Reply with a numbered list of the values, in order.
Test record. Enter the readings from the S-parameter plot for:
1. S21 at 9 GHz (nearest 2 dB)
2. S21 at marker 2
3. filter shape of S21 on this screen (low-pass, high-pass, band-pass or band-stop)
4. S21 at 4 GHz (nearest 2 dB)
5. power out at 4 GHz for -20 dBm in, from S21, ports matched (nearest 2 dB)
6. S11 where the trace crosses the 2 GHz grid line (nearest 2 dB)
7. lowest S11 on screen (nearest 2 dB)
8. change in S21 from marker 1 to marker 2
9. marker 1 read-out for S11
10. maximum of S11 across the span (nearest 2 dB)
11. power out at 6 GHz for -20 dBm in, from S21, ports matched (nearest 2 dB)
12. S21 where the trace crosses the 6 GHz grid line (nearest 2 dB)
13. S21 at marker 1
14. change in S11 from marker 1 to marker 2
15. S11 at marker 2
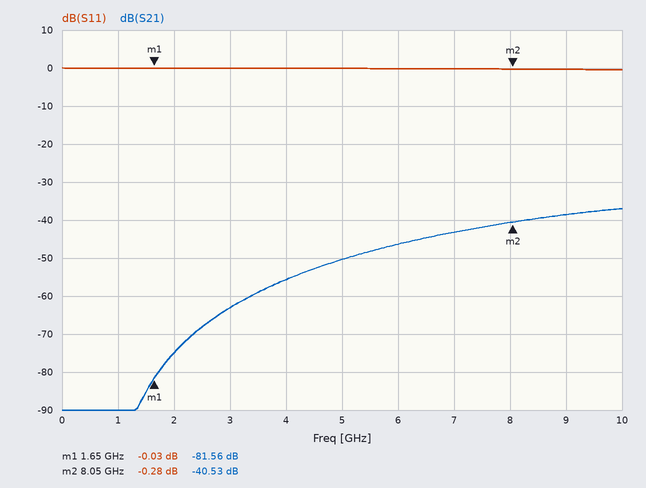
1. -38 dB
2. -40.53 dB
3. high-pass
4. -56 dB
5. -76 dBm
6. 0 dB
7. 0 dB
8. 41.03 dB
9. -0.03 dB
10. 0 dB
11. -66 dBm
12. -46 dB
13. -81.56 dB
14. -0.25 dB
15. -0.28 dB
